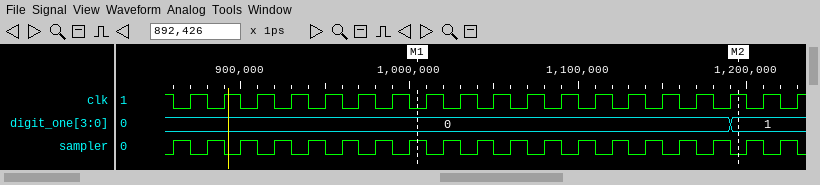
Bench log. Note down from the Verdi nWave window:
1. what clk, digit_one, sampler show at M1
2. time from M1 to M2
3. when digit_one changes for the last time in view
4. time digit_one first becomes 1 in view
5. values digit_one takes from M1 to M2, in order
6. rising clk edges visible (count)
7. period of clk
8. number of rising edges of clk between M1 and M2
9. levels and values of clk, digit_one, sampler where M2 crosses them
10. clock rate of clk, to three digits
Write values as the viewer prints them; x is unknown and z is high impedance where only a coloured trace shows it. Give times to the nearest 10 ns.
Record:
clk=0, digit_one=0, sampler=1
190 ns
1190 ns
1190 ns
0, 1
19
20 ns
10
clk=1, digit_one=1, sampler=0
50.0 MHz
